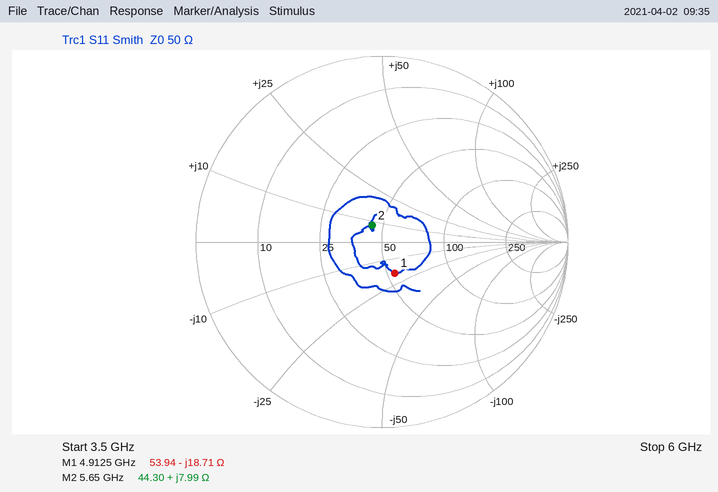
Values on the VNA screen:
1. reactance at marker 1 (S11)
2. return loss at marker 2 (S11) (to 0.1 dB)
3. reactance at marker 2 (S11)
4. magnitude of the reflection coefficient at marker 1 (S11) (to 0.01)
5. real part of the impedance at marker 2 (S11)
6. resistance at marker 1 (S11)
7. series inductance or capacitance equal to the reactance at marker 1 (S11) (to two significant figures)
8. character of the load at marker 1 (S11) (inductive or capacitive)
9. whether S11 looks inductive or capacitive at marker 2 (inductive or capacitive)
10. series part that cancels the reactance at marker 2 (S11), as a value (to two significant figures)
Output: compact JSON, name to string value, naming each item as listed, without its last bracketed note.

{"reactance at marker 1": "-18.71 Ω", "return loss at marker 2 (S11)": "19.7 dB", "reactance at marker 2": "+7.99 Ω", "magnitude of the reflection coefficient at marker 1 (S11)": "0.18", "real part of the impedance at marker 2": "44.30 Ω", "resistance at marker 1": "53.94 Ω", "series inductance or capacitance equal to the reactance at marker 1 (S11)": "1.7 pF", "character of the load at marker 1 (S11)": "capacitive", "whether S11 looks inductive or capacitive at marker 2": "inductive", "series part that cancels the reactance at marker 2 (S11), as a value": "3.5 pF"}
